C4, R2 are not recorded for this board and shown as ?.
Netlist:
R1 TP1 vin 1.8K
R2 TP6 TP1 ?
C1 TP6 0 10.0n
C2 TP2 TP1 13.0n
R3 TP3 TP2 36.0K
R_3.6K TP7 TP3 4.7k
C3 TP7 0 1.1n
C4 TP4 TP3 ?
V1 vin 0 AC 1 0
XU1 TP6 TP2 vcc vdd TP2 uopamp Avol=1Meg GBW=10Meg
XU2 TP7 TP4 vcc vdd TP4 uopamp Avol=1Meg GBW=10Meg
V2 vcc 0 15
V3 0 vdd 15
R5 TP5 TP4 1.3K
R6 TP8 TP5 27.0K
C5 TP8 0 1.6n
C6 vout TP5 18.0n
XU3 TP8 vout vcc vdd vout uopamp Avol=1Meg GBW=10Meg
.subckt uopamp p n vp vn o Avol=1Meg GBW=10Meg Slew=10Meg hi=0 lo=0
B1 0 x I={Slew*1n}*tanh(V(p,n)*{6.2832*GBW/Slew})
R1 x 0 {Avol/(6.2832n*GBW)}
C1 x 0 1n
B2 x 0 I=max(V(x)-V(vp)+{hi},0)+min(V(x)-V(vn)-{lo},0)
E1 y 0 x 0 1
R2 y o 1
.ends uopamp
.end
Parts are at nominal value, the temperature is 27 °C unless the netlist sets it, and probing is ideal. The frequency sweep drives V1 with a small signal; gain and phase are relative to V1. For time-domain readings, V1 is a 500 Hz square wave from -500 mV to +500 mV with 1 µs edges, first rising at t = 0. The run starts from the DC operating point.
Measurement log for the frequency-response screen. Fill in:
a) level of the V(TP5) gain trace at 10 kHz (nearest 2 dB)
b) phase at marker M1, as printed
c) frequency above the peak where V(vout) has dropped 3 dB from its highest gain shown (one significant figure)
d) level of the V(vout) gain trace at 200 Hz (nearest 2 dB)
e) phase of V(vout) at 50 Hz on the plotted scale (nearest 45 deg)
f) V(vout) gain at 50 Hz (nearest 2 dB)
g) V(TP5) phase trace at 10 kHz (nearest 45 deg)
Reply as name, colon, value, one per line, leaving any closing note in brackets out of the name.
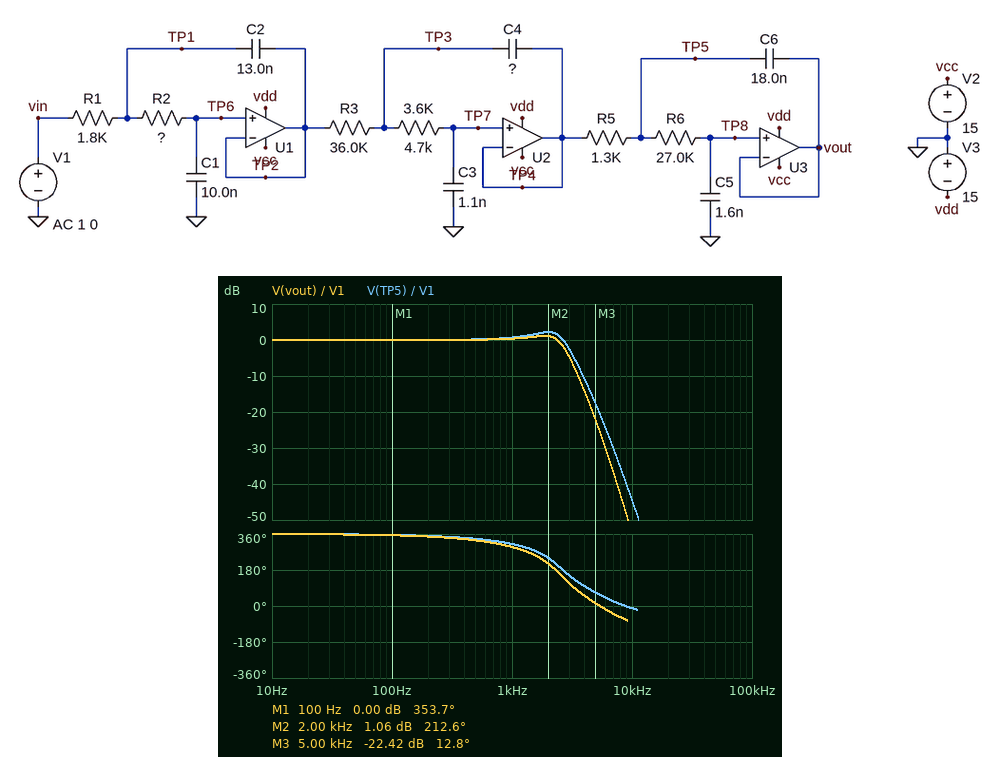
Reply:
level of the V(TP5) gain trace at 10 kHz: -44 dB
phase at marker M1, as printed: 353.7 deg
frequency above the peak where V(vout) has dropped 3 dB from its highest gain shown: 3 kHz
level of the V(vout) gain trace at 200 Hz: 0 dB
phase of V(vout) at 50 Hz on the plotted scale: 360 deg
V(vout) gain at 50 Hz: 0 dB
V(TP5) phase trace at 10 kHz: 0 deg
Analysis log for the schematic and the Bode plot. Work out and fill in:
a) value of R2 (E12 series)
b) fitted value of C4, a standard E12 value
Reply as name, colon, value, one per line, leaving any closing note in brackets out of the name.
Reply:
value of R2: 6.8 kΩ
fitted value of C4, a standard E12 value: 22 nF
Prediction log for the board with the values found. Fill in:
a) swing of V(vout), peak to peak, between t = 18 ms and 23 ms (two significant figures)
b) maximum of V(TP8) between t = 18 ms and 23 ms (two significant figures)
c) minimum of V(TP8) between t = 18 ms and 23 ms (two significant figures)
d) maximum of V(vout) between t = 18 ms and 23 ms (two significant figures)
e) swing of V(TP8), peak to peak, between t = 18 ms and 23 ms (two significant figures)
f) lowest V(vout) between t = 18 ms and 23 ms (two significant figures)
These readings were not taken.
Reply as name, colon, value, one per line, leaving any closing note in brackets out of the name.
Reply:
swing of V(vout), peak to peak, between t = 18 ms and 23 ms: 1.4 V
maximum of V(TP8) between t = 18 ms and 23 ms: 680 mV
minimum of V(TP8) between t = 18 ms and 23 ms: -680 mV
maximum of V(vout) between t = 18 ms and 23 ms: 680 mV
swing of V(TP8), peak to peak, between t = 18 ms and 23 ms: 1.4 V
lowest V(vout) between t = 18 ms and 23 ms: -680 mV
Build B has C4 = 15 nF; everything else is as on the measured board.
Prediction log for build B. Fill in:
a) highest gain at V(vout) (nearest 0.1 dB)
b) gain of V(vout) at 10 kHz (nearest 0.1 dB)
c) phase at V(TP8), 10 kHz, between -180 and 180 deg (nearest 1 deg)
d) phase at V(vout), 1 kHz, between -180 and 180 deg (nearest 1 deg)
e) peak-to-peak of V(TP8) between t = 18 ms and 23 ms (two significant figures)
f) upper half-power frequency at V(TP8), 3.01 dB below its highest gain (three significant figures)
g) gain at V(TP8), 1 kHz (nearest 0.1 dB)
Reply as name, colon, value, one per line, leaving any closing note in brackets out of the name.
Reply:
highest gain at V(vout): 0 dB
gain of V(vout) at 10 kHz: -50.3 dB
phase at V(TP8), 10 kHz, between -180 and 180 deg: -75 deg
phase at V(vout), 1 kHz, between -180 and 180 deg: -64 deg
peak-to-peak of V(TP8) between t = 18 ms and 23 ms: 1.2 V
upper half-power frequency at V(TP8), 3.01 dB below its highest gain: 2.89 kHz
gain at V(TP8), 1 kHz: -0.1 dB
